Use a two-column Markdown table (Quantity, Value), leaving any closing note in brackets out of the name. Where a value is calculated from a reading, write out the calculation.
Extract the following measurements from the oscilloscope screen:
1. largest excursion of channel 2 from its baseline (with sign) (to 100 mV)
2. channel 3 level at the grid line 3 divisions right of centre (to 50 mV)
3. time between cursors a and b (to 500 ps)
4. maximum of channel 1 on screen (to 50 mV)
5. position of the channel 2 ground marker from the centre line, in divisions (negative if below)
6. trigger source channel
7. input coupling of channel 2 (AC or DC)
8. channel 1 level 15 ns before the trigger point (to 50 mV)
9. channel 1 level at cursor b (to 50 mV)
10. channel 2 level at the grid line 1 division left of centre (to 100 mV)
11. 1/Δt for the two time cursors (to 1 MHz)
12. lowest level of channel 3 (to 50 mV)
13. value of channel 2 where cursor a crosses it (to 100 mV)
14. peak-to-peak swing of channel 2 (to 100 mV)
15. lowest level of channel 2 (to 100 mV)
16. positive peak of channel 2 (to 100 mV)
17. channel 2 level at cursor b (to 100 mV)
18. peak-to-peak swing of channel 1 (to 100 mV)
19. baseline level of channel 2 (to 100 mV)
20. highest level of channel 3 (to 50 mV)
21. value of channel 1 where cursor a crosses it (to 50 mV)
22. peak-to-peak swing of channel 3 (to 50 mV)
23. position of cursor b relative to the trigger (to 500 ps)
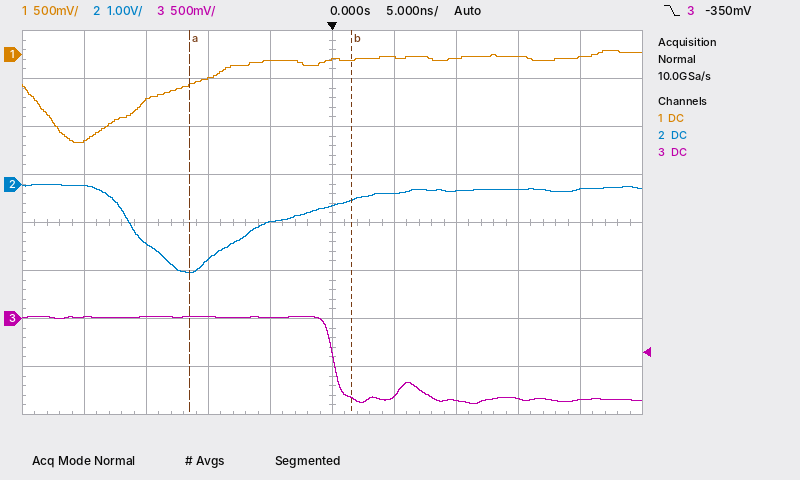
| Quantity | Value |
|---|---|
| largest excursion of channel 2 from its baseline (with sign) | -1.8 V − (-100 mV) = -1.7 V |
| channel 3 level at the grid line 3 divisions right of centre | -850 mV |
| time between cursors a and b | 13.0 ns |
| maximum of channel 1 on screen | 50 mV |
| position of the channel 2 ground marker from the centre line, in divisions | +0.8 div |
| trigger source channel | channel 3 |
| input coupling of channel 2 | DC |
| channel 1 level 15 ns before the trigger point | -500 mV |
| channel 1 level at cursor b | -50 mV |
| channel 2 level at the grid line 1 division left of centre | -800 mV |
| 1/Δt for the two time cursors | 1 / 13.0 ns ≈ 77 MHz |
| lowest level of channel 3 | -900 mV |
| value of channel 2 where cursor a crosses it | -1.8 V |
| peak-to-peak swing of channel 2 | 0.0 V − (-1.8 V) = 1.8 V |
| lowest level of channel 2 | -1.8 V |
| positive peak of channel 2 | 0.0 V |
| channel 2 level at cursor b | -300 mV |
| peak-to-peak swing of channel 1 | 1.00 V |
| baseline level of channel 2 | -100 mV |
| highest level of channel 3 | 0 mV |
| value of channel 1 where cursor a crosses it | -300 mV |
| peak-to-peak swing of channel 3 | 0 mV − (-900 mV) = 900 mV |
| position of cursor b relative to the trigger | +1.5 ns |
